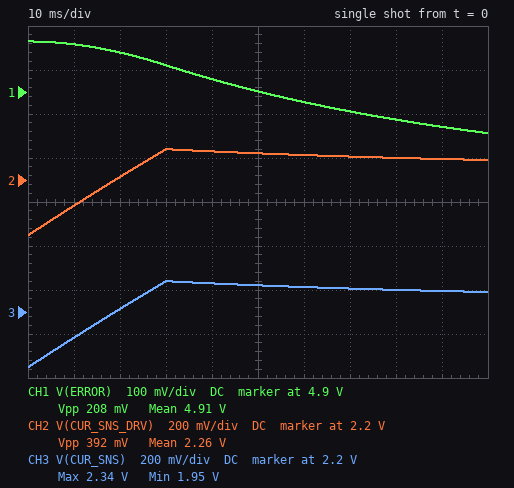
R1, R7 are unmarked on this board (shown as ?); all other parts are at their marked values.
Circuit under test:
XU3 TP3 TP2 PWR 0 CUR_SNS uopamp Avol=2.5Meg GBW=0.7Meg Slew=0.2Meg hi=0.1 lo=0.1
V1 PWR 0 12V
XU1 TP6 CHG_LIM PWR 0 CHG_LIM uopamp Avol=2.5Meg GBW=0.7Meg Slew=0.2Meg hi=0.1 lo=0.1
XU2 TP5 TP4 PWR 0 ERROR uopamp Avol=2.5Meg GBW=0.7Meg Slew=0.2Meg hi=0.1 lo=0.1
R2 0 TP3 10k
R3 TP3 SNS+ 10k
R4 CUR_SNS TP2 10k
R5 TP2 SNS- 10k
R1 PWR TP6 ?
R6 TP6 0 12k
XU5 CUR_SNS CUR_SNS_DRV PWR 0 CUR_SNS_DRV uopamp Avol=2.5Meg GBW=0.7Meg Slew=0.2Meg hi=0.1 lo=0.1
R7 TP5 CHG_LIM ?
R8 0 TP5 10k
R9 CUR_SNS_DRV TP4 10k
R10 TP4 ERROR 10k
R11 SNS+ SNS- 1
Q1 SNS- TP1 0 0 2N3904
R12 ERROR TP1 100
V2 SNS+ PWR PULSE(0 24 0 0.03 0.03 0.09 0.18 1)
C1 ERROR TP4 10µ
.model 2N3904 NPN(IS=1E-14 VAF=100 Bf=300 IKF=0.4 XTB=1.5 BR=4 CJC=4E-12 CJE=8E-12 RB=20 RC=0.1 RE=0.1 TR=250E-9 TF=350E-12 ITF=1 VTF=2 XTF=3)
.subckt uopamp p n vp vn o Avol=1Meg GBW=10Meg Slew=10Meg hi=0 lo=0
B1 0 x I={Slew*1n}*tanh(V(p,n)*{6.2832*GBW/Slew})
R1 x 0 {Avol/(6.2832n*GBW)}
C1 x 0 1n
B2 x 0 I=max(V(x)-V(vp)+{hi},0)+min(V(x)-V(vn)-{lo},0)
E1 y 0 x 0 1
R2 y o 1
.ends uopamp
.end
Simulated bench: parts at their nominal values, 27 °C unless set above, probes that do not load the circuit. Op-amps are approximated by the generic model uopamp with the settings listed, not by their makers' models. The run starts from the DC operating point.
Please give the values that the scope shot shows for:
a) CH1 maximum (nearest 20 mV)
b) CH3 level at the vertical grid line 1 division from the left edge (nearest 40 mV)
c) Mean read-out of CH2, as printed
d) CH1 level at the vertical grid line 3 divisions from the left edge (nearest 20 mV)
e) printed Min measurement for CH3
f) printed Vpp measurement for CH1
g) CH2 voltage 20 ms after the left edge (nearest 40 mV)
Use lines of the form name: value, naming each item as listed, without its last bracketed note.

CH1 maximum: 5.02 V
CH3 level at the vertical grid line 1 division from the left edge: 2.08 V
Mean read-out of CH2, as printed: 2.26 V
CH1 level at the vertical grid line 3 divisions from the left edge: 4.96 V
printed Min measurement for CH3: 1.95 V
printed Vpp measurement for CH1: 208 mV
CH2 voltage 20 ms after the left edge: 2.20 V
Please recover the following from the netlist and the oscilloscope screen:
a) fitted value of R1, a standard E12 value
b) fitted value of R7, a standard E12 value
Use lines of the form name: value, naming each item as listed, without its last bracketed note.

fitted value of R1, a standard E12 value: 6.8 kΩ
fitted value of R7, a standard E12 value: 12 kΩ
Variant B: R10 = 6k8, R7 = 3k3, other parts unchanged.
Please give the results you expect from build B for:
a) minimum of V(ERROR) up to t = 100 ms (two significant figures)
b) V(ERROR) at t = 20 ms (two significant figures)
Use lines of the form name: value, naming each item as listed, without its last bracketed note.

minimum of V(ERROR) up to t = 100 ms: 7.7 V
V(ERROR) at t = 20 ms: 7.9 V
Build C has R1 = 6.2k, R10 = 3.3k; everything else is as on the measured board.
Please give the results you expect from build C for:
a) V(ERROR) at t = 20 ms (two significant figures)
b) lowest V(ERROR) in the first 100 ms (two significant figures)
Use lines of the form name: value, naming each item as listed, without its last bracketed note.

V(ERROR) at t = 20 ms: 4.2 V
lowest V(ERROR) in the first 100 ms: 4.1 V
